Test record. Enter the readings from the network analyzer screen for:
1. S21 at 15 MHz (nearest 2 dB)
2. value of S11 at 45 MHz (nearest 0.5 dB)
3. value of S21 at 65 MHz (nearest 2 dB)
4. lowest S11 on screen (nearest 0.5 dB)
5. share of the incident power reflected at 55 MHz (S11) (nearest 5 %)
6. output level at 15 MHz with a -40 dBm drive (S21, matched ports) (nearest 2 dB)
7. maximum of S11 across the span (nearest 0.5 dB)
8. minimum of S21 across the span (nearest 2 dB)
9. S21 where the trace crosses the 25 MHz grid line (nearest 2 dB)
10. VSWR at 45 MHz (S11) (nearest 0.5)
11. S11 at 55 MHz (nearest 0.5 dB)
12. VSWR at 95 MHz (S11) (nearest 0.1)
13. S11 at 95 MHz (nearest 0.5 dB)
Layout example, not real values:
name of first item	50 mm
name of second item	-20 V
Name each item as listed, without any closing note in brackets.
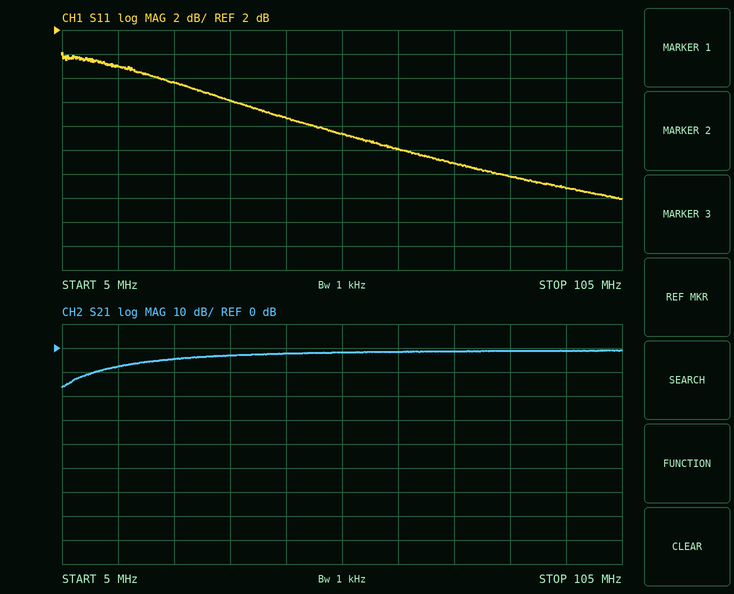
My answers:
S21 at 15 MHz	-8 dB
value of S11 at 45 MHz	-5.5 dB
value of S21 at 65 MHz	-2 dB
lowest S11 on screen	-12.0 dB
share of the incident power reflected at 55 MHz (S11)	20 %
output level at 15 MHz with a -40 dBm drive (S21, matched ports)	-48 dBm
maximum of S11 across the span	0.0 dB
minimum of S21 across the span	-16 dB
S21 where the trace crosses the 25 MHz grid line	-4 dB
VSWR at 45 MHz (S11)	3.5
S11 at 55 MHz	-6.5 dB
VSWR at 95 MHz (S11)	1.8
S11 at 95 MHz	-11.0 dB
